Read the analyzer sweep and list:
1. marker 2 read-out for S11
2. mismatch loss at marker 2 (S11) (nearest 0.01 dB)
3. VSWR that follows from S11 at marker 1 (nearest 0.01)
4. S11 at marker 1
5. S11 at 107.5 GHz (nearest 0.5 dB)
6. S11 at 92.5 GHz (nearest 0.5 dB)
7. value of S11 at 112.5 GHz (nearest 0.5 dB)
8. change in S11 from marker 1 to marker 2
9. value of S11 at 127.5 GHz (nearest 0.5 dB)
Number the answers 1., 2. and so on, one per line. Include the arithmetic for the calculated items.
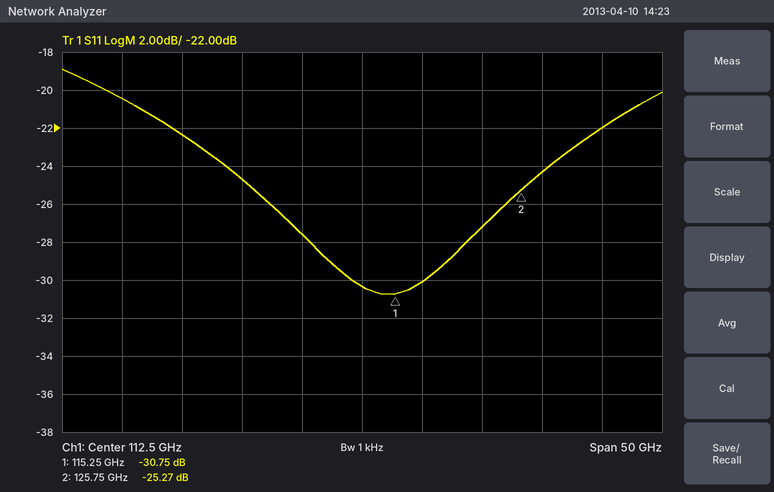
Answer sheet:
1. -25.27 dB
2. −10 log10(1 − 10^(-25.27/10)) ≈ 0.01 dB
3. (1 + 0.0290)/(1 − 0.0290) ≈ 1.06
4. -30.75 dB
5. -27.5 dB
6. -20.5 dB
7. -30.5 dB
8. -25.27 − (-30.75) = 5.48 dB
9. -24.5 dB
